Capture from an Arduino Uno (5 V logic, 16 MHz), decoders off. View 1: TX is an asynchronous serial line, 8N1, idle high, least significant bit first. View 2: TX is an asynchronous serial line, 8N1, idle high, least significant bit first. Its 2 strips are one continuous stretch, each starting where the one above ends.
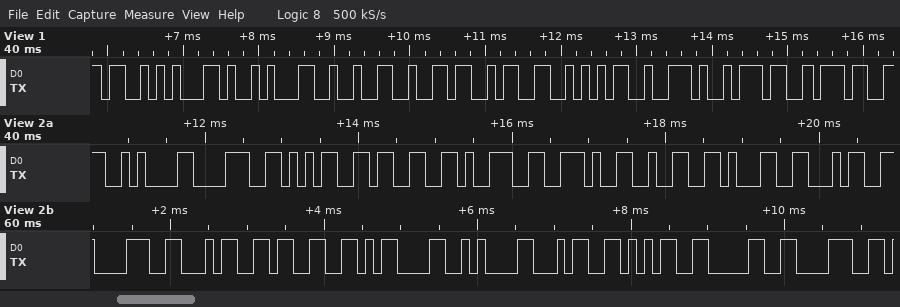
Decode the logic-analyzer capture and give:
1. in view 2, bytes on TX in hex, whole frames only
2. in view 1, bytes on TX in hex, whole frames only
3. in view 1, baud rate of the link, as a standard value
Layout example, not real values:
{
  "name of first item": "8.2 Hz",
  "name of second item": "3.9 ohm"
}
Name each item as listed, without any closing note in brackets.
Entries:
{
  "in view 2, bytes on TX in hex, whole frames only": "0x0A 0x38 0x35 0x33 0x39 0x2E 0x32 0x31 0x34 0x38 0x34 0x33 0x0D 0x0A 0x34 0x35 0x30 0x38",
  "in view 1, bytes on TX in hex, whole frames only": "53 2C 31 32 36 33 35 2E 37 37",
  "in view 1, baud rate of the link, as a standard value": "9600 baud"
}
